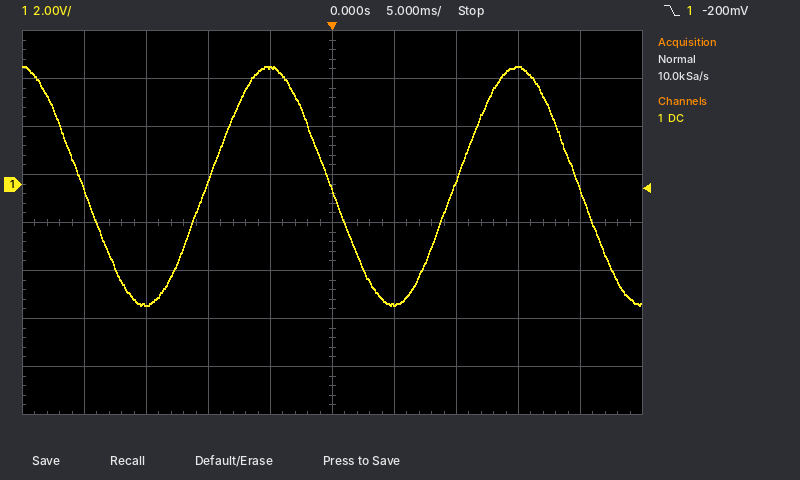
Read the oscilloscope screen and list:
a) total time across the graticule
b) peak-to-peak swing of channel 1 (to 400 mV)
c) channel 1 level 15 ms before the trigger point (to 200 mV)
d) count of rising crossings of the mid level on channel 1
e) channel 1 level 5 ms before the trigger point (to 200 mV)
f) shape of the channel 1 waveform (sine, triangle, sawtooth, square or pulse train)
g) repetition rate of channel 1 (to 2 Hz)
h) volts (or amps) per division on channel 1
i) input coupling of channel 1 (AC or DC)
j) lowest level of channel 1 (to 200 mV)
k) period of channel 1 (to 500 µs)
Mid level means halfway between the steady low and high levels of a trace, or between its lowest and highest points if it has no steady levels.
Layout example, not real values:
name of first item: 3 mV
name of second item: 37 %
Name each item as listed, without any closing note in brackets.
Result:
total time across the graticule: 50 ms
peak-to-peak swing of channel 1: 10.0 V
channel 1 level 15 ms before the trigger point: -5.0 V
count of rising crossings of the mid level on channel 1: 2
channel 1 level 5 ms before the trigger point: 4.8 V
shape of the channel 1 waveform: sine
repetition rate of channel 1: 50 Hz
volts (or amps) per division on channel 1: 2 V
input coupling of channel 1: DC
lowest level of channel 1: -5.0 V
period of channel 1: 20.0 ms
